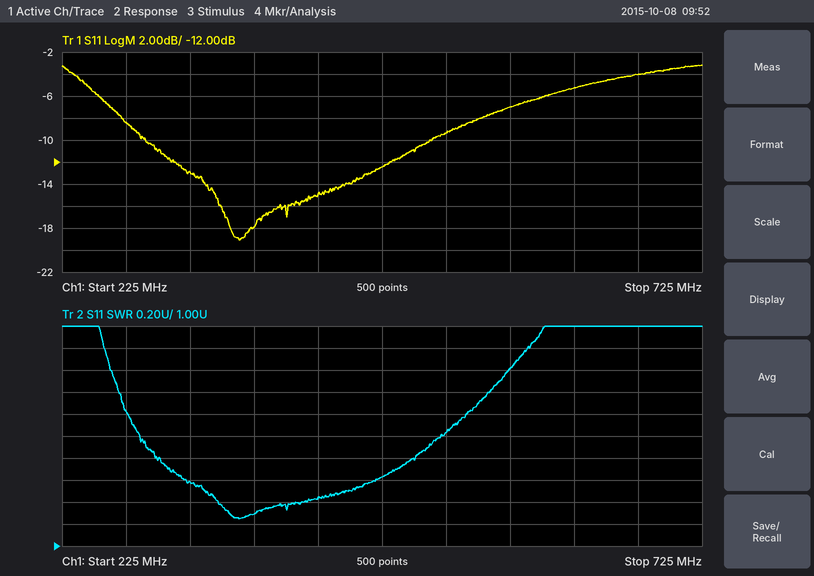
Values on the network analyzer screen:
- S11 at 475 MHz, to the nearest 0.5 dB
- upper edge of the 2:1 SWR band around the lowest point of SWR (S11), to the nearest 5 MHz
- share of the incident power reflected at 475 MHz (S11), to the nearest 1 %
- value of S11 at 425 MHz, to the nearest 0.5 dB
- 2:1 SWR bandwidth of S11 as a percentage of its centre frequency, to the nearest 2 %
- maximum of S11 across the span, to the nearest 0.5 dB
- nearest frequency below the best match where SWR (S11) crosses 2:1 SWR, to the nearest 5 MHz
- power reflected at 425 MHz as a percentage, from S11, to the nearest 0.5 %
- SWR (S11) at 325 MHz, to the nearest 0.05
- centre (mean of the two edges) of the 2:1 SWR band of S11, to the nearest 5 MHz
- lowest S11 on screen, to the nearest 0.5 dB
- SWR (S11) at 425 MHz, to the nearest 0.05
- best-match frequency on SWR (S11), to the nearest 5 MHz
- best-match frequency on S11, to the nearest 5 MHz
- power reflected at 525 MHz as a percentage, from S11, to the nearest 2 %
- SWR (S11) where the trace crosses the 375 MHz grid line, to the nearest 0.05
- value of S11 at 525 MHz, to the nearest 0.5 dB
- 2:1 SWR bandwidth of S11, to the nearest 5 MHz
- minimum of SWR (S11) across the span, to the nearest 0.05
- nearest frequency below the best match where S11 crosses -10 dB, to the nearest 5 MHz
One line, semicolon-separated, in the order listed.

-12.5 dB; 520 MHz; 6 %; -15.0 dB; 58 %; -3.0 dB; 285 MHz; 3.0 %; 1.60; 405 MHz; -19.0 dB; 1.45; 365 MHz; 365 MHz; 12 %; 1.30; -9.5 dB; 235 MHz; 1.25; 290 MHz
